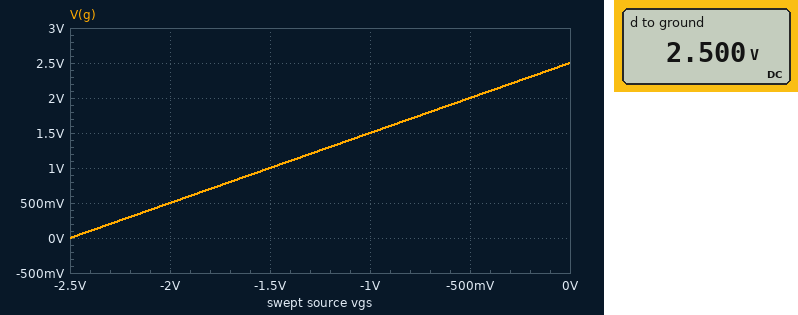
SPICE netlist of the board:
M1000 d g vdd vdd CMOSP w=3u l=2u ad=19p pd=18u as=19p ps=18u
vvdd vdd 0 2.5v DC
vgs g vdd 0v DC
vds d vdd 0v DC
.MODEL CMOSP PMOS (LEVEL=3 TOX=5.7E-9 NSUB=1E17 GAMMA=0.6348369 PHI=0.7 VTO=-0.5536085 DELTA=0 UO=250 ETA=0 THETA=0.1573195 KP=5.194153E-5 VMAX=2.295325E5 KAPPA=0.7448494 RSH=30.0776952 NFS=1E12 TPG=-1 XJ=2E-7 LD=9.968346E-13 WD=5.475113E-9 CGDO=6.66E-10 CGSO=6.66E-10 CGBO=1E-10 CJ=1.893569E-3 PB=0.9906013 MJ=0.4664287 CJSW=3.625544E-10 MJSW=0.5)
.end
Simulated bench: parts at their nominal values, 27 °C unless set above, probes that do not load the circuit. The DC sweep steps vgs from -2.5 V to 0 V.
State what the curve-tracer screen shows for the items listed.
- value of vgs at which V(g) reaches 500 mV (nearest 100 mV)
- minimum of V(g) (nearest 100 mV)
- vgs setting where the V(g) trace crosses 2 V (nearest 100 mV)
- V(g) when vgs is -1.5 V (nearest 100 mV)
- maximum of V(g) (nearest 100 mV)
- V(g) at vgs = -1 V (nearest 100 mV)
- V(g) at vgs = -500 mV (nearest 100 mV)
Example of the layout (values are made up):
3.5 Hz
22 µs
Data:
-2.0 V
0 V
-500 mV
1.0 V
2.5 V
1.5 V
2.0 V
